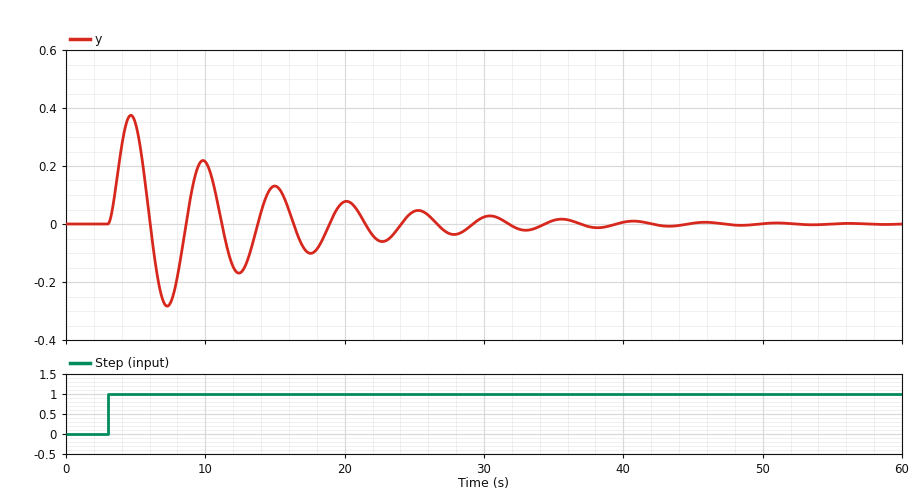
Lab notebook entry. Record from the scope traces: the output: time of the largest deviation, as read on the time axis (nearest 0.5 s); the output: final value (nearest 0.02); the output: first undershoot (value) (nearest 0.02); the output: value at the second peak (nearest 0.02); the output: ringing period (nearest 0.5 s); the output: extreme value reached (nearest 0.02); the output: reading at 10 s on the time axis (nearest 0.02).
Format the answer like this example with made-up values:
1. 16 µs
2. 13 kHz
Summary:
1. 4.5 s
2. 0.00
3. -0.28
4. 0.22
5. 5.0 s
6. 0.38
7. 0.22
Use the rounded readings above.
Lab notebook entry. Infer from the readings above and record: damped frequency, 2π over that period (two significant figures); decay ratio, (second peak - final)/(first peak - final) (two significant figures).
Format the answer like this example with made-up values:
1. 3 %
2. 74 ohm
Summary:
1. 1.3 rad/s
2. 0.58
